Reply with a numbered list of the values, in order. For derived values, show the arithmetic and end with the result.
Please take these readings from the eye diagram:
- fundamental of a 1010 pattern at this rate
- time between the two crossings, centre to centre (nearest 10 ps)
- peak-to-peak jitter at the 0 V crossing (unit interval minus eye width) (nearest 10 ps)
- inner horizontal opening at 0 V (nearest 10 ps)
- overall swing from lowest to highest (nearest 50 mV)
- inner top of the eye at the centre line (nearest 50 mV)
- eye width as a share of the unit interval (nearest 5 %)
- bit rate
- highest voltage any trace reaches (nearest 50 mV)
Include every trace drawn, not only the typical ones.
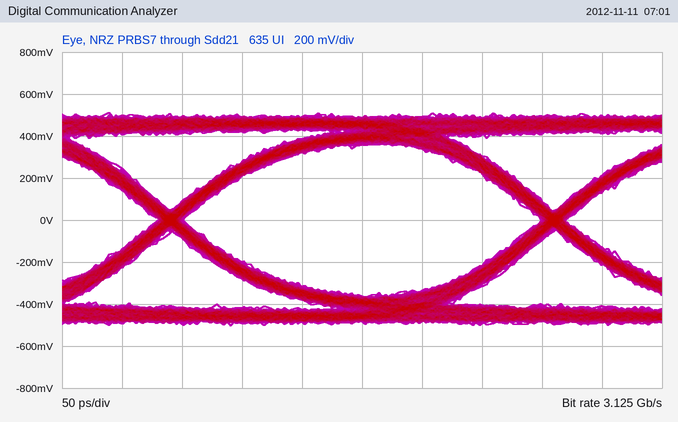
1. 1.5625 GHz
2. 320 ps
3. 20 ps
4. 300 ps
5. 1.00 V
6. 350 mV
7. 300 ps / 320 ps ≈ 93.8 %, so 95 % to the nearest 5 %
8. 3.125 Gb/s
9. 500 mV
